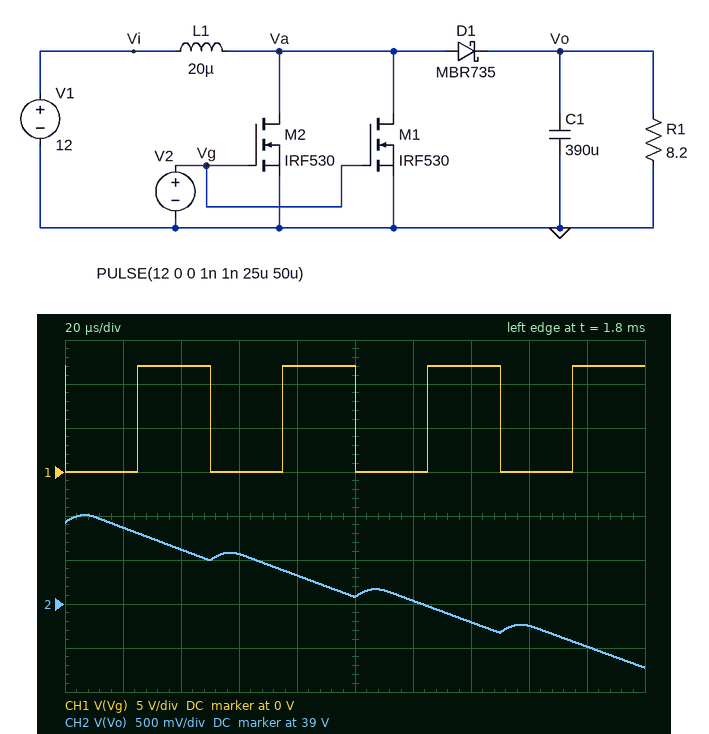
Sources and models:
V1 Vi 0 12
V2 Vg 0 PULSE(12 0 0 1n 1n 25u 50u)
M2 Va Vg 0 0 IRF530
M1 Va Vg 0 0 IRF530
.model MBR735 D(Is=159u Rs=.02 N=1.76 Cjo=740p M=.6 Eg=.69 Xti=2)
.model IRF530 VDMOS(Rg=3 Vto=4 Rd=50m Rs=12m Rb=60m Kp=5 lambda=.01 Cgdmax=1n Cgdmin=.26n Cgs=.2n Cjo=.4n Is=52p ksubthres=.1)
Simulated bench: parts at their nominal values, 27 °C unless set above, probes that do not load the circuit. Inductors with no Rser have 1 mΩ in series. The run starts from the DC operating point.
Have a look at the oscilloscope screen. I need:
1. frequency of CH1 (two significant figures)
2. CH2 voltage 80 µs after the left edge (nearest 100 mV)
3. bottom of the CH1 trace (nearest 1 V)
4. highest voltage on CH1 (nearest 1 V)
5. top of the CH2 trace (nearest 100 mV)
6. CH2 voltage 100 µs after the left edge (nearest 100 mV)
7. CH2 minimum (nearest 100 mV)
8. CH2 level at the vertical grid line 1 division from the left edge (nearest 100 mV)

20 kHz
39.3 V
0 V
12 V
40.0 V
39.1 V
38.3 V
39.9 V
